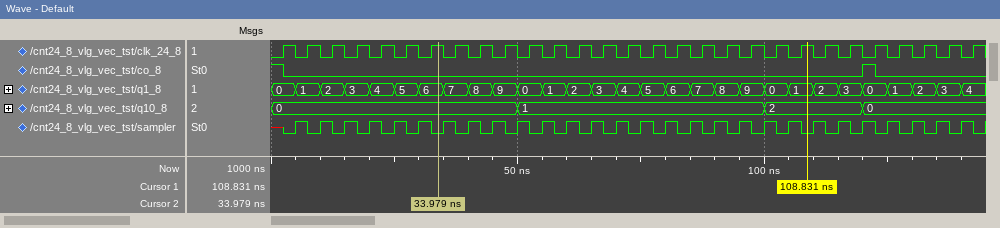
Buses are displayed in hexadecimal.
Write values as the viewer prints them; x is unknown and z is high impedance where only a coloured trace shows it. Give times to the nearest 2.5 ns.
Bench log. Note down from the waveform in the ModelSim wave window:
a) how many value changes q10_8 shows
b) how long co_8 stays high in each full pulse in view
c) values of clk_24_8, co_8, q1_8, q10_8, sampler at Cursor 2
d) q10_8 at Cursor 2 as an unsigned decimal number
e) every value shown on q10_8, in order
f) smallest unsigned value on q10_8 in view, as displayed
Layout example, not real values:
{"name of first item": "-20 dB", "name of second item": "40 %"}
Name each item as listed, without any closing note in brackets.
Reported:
{"how many value changes q10_8 shows": "3", "how long co_8 stays high in each full pulse in view": "2.5 ns", "values of clk_24_8, co_8, q1_8, q10_8, sampler at Cursor 2": "clk_24_8=1, co_8=0, q1_8=6, q10_8=0, sampler=0", "q10_8 at Cursor 2 as an unsigned decimal number": "0", "every value shown on q10_8, in order": "0, 1, 2, 0", "smallest unsigned value on q10_8 in view, as displayed": "0"}
